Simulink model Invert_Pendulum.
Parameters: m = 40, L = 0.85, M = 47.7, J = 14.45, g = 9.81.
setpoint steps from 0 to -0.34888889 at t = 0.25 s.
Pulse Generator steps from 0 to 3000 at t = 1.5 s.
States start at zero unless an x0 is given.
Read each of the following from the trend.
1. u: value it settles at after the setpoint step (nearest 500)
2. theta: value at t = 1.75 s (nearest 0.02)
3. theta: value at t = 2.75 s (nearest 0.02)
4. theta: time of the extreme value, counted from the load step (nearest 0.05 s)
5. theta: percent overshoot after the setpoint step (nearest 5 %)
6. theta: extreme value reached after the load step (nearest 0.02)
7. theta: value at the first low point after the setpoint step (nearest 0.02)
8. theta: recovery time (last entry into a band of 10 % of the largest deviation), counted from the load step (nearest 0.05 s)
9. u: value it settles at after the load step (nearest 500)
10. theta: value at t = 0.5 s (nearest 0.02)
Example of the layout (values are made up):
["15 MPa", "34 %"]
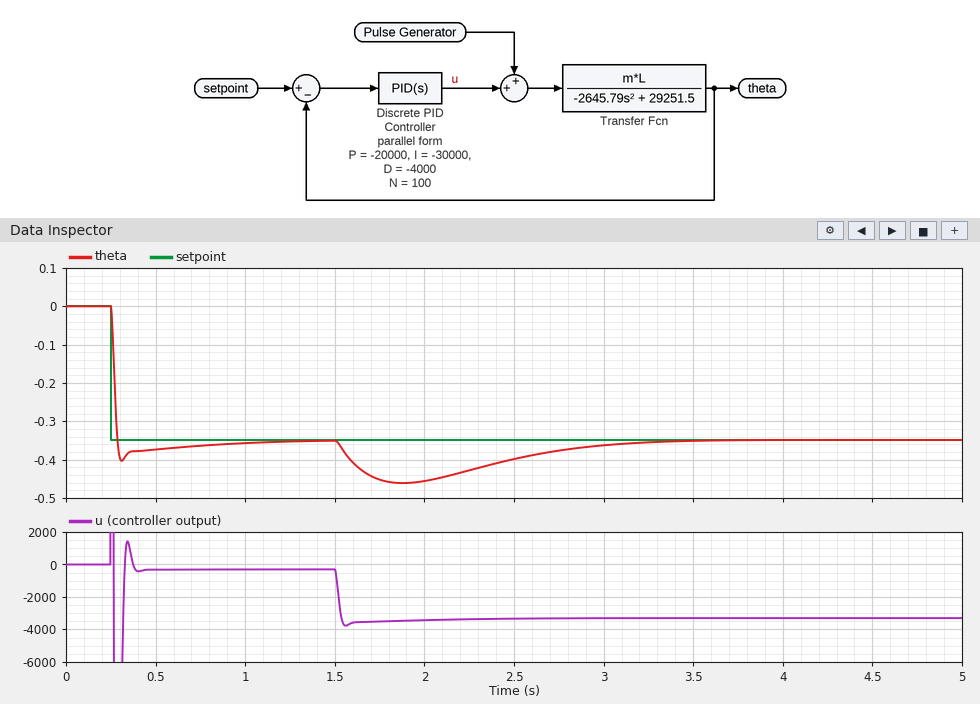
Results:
["-500", "-0.46", "-0.38", "0.40 s", "15 %", "-0.46", "-0.40", "1.55 s", "-3500", "-0.38"]
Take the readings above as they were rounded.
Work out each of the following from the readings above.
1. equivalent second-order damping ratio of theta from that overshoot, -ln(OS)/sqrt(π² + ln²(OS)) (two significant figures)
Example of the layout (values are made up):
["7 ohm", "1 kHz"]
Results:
["0.52"]
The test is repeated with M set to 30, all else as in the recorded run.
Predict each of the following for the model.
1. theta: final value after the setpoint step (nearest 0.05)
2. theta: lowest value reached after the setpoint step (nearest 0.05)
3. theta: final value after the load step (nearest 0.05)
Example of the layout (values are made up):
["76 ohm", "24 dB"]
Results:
["-0.35", "-0.40", "-0.35"]
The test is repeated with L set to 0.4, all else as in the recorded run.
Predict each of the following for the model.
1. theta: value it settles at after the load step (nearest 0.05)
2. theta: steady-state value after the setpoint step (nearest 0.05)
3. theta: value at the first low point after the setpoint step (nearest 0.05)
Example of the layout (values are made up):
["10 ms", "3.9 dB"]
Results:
["-0.35", "-0.35", "-0.40"]
